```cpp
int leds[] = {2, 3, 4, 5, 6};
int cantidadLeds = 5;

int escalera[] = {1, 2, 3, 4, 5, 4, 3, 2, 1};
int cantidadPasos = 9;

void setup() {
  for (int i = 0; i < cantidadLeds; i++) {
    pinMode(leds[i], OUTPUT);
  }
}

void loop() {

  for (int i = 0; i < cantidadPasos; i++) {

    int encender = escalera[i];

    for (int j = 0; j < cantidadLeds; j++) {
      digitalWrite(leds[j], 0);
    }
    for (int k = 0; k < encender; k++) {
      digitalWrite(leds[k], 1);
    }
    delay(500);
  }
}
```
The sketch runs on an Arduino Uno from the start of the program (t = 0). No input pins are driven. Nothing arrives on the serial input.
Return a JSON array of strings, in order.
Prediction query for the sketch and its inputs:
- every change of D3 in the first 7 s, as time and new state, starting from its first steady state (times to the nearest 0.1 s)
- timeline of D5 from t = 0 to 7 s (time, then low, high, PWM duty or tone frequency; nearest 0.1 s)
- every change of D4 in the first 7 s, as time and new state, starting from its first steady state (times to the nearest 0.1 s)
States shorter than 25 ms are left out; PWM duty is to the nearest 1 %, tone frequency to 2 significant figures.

["0 s low; 0.5 s high; 4 s low; 5 s high", "0 s low; 1.5 s high; 3 s low; 6 s high", "0 s low; 1 s high; 3.5 s low; 5.5 s high"]
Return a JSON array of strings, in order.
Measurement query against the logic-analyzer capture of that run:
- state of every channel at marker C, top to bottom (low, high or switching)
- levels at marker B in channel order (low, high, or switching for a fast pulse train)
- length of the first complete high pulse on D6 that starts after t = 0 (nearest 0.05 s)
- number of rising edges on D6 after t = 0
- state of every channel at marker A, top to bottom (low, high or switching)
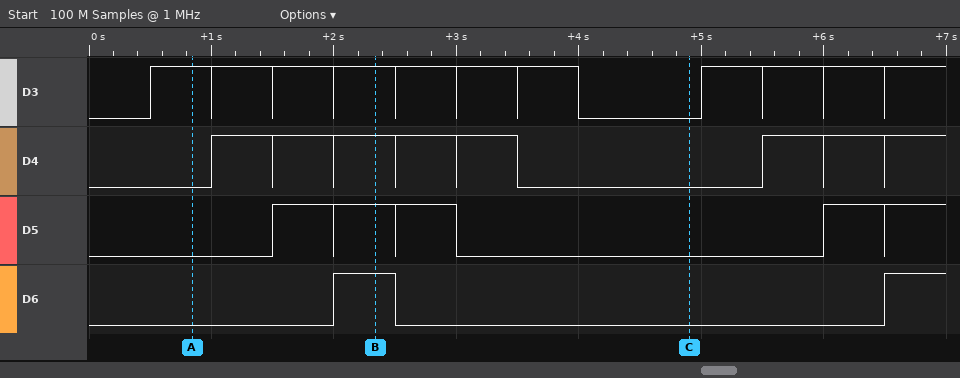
["D3 low, D4 low, D5 low, D6 low", "D3 high, D4 high, D5 high, D6 high", "0.50 s", "2", "D3 high, D4 low, D5 low, D6 low"]
